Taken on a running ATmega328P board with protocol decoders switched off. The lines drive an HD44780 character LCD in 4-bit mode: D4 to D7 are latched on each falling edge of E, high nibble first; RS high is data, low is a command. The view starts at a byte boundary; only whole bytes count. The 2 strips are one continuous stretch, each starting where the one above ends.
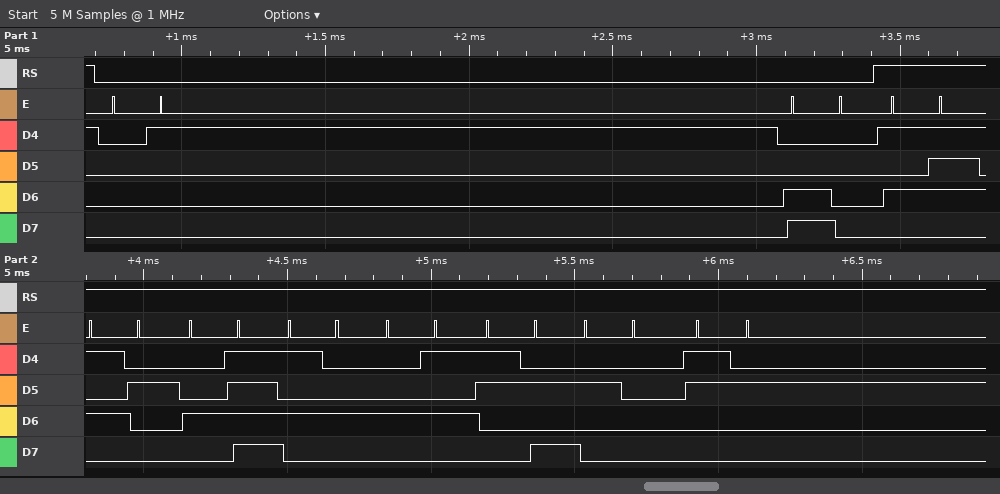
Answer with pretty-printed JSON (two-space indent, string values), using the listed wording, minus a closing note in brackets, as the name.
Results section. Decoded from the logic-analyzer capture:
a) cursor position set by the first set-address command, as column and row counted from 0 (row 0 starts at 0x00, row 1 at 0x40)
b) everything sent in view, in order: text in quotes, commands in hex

{
  "cursor position set by the first set-address command, as column and row counted from 0": "column 0, row 1",
  "everything sent in view, in order: text in quotes, commands in hex": "0x01 0xC0 \"WROTE: 2\""
}
